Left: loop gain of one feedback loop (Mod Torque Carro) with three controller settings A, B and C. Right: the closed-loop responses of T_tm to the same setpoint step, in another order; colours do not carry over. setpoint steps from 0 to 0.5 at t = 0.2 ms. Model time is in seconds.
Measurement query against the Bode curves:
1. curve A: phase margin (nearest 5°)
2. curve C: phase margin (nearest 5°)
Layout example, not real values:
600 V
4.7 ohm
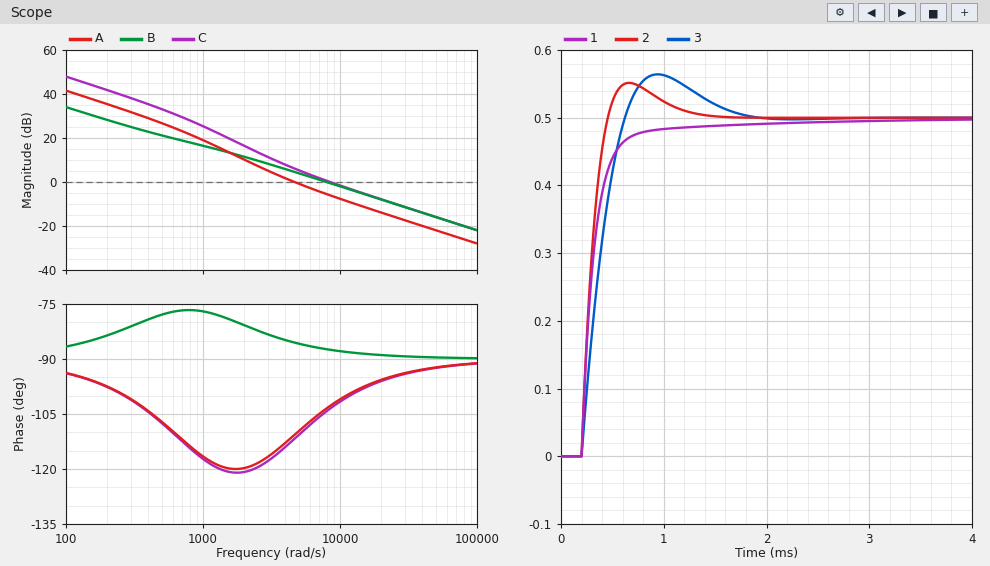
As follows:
70°
75°
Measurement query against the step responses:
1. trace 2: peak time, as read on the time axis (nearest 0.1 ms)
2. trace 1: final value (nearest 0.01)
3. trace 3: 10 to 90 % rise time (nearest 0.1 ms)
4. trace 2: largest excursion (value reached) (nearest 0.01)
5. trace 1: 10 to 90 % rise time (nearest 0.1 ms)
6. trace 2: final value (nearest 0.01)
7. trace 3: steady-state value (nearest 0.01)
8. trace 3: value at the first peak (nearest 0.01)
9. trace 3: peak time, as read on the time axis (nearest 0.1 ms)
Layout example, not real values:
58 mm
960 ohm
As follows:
0.7 ms
0.50
0.3 ms
0.55
0.3 ms
0.50
0.50
0.56
0.9 ms
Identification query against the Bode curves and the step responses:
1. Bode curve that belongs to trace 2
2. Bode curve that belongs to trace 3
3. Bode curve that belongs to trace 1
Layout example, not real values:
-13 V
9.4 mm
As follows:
C
A
B
